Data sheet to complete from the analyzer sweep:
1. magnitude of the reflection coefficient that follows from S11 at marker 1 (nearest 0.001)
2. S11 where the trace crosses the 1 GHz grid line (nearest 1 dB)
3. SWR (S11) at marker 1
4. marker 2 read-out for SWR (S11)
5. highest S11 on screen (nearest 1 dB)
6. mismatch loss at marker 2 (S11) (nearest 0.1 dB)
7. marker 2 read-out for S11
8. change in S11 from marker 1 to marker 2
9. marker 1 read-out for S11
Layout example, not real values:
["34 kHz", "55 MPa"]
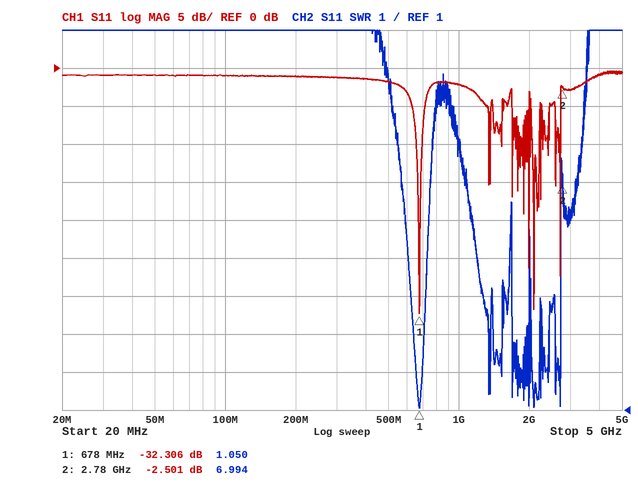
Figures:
["0.024", "-2 dB", "1.050", "6.994", "0 dB", "3.6 dB", "-2.501 dB", "29.805 dB", "-32.306 dB"]
